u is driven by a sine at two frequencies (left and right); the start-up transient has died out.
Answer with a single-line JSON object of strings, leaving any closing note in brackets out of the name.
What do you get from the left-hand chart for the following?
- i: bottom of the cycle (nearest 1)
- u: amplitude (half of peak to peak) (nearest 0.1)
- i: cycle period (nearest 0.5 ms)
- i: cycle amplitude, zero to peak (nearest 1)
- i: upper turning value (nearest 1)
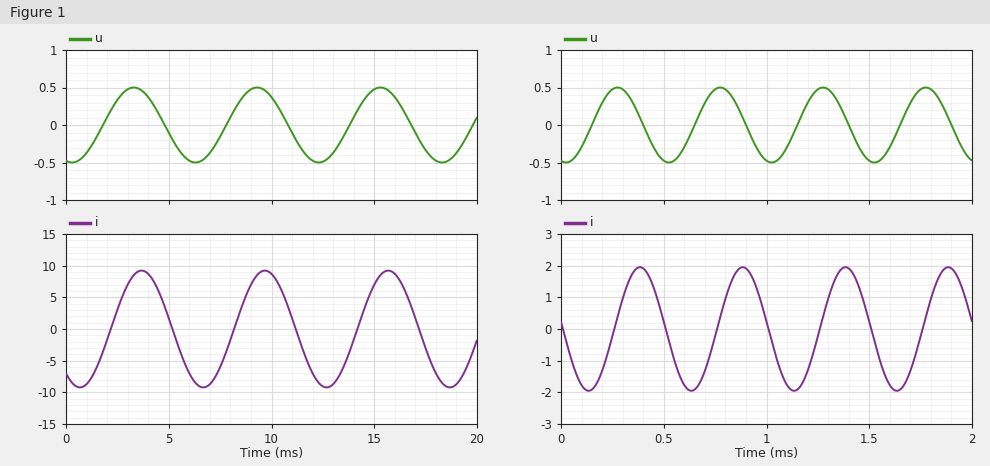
{"i: bottom of the cycle": "-9", "u: amplitude (half of peak to peak)": "0.5", "i: cycle period": "6.0 ms", "i: cycle amplitude, zero to peak": "9", "i: upper turning value": "9"}
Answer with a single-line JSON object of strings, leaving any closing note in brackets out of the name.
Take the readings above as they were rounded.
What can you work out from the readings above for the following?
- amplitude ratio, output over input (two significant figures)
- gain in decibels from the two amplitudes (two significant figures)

{"amplitude ratio, output over input": "18", "gain in decibels from the two amplitudes": "25 dB"}
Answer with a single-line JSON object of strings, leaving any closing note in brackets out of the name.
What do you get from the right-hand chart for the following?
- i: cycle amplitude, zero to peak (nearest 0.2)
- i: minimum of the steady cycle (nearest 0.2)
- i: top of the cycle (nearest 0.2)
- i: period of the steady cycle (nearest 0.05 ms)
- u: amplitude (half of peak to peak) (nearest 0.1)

{"i: cycle amplitude, zero to peak": "2.0", "i: minimum of the steady cycle": "-2.0", "i: top of the cycle": "2.0", "i: period of the steady cycle": "0.50 ms", "u: amplitude (half of peak to peak)": "0.5"}
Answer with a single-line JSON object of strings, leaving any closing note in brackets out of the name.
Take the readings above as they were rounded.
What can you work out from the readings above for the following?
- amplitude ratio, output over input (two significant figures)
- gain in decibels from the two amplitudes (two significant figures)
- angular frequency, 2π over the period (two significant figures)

{"amplitude ratio, output over input": "4.0", "gain in decibels from the two amplitudes": "12 dB", "angular frequency, 2π over the period": "13 rad/ms"}
